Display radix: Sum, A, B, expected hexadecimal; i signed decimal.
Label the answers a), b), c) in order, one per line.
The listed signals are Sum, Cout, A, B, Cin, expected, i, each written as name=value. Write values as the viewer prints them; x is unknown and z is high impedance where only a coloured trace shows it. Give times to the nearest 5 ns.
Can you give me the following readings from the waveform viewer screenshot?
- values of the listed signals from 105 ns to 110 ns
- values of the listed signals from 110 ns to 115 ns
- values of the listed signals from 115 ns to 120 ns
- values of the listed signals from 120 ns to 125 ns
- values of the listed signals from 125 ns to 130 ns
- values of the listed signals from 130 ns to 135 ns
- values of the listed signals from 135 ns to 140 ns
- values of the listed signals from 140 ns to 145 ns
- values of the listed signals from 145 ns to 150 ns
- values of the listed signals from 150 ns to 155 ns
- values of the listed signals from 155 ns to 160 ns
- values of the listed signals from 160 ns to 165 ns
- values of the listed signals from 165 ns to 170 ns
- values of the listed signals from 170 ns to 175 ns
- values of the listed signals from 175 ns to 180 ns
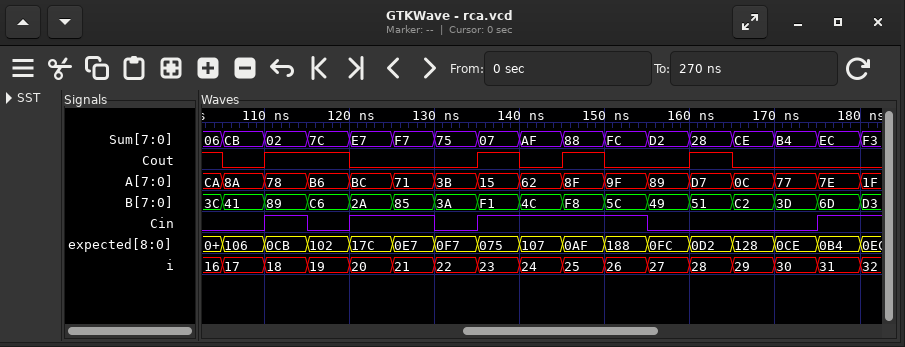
a) Sum=CB, Cout=0, A=8A, B=41, Cin=0, expected=106, i=17
b) Sum=02, Cout=1, A=78, B=89, Cin=1, expected=0CB, i=18
c) Sum=7C, Cout=1, A=B6, B=C6, Cin=0, expected=102, i=19
d) Sum=E7, Cout=0, A=BC, B=2A, Cin=1, expected=17C, i=20
e) Sum=F7, Cout=0, A=71, B=85, Cin=1, expected=0E7, i=21
f) Sum=75, Cout=0, A=3B, B=3A, Cin=0, expected=0F7, i=22
g) Sum=07, Cout=1, A=15, B=F1, Cin=1, expected=075, i=23
h) Sum=AF, Cout=0, A=62, B=4C, Cin=1, expected=107, i=24
i) Sum=88, Cout=1, A=8F, B=F8, Cin=1, expected=0AF, i=25
j) Sum=FC, Cout=0, A=9F, B=5C, Cin=1, expected=188, i=26
k) Sum=D2, Cout=0, A=89, B=49, Cin=0, expected=0FC, i=27
l) Sum=28, Cout=1, A=D7, B=51, Cin=0, expected=0D2, i=28
m) Sum=CE, Cout=0, A=0C, B=C2, Cin=0, expected=128, i=29
n) Sum=B4, Cout=0, A=77, B=3D, Cin=0, expected=0CE, i=30
o) Sum=EC, Cout=0, A=7E, B=6D, Cin=1, expected=0B4, i=31
